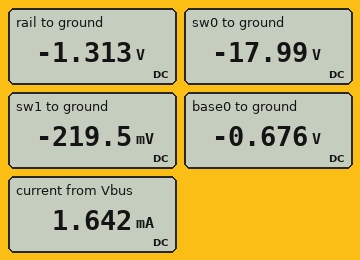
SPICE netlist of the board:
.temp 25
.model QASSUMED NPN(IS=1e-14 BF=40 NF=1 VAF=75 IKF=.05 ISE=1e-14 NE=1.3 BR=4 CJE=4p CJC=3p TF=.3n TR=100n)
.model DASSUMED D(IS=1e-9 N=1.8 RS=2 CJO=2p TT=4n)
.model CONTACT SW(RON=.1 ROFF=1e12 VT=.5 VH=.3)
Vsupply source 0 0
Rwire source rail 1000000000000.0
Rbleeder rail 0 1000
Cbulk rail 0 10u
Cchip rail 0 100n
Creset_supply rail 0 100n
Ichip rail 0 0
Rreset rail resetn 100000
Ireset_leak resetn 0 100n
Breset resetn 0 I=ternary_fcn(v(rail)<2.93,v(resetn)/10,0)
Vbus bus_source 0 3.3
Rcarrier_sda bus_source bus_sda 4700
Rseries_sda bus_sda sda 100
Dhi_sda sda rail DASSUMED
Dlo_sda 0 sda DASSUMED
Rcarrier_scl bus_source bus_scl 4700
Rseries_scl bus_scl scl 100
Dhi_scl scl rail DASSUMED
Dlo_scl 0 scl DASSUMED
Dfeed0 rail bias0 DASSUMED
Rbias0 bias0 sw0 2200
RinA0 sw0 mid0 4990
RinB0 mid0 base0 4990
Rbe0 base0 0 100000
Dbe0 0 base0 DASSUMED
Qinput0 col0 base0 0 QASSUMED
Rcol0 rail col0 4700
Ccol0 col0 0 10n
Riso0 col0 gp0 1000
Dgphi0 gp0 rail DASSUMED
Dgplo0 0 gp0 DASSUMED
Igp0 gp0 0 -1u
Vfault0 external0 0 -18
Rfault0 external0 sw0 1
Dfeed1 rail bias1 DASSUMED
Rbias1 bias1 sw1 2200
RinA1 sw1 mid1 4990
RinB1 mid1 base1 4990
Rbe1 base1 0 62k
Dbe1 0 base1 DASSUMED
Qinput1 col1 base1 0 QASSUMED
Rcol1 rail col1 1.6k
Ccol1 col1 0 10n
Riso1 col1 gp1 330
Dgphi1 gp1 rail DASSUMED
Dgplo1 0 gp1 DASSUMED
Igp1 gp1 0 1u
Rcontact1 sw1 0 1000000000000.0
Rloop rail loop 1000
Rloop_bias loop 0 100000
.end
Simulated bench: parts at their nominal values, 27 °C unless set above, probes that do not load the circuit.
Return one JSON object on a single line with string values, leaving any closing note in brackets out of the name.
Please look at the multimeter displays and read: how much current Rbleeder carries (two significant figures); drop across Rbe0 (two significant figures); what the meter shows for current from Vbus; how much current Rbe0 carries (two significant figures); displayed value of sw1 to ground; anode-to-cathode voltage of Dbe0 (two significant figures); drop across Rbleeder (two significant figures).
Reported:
{"how much current Rbleeder carries": "1.3 mA", "drop across Rbe0": "680 mV", "what the meter shows for current from Vbus": "1.642 mA", "how much current Rbe0 carries": "6.8 µA", "displayed value of sw1 to ground": "-219.5 mV", "anode-to-cathode voltage of Dbe0": "680 mV", "drop across Rbleeder": "1.3 V"}
